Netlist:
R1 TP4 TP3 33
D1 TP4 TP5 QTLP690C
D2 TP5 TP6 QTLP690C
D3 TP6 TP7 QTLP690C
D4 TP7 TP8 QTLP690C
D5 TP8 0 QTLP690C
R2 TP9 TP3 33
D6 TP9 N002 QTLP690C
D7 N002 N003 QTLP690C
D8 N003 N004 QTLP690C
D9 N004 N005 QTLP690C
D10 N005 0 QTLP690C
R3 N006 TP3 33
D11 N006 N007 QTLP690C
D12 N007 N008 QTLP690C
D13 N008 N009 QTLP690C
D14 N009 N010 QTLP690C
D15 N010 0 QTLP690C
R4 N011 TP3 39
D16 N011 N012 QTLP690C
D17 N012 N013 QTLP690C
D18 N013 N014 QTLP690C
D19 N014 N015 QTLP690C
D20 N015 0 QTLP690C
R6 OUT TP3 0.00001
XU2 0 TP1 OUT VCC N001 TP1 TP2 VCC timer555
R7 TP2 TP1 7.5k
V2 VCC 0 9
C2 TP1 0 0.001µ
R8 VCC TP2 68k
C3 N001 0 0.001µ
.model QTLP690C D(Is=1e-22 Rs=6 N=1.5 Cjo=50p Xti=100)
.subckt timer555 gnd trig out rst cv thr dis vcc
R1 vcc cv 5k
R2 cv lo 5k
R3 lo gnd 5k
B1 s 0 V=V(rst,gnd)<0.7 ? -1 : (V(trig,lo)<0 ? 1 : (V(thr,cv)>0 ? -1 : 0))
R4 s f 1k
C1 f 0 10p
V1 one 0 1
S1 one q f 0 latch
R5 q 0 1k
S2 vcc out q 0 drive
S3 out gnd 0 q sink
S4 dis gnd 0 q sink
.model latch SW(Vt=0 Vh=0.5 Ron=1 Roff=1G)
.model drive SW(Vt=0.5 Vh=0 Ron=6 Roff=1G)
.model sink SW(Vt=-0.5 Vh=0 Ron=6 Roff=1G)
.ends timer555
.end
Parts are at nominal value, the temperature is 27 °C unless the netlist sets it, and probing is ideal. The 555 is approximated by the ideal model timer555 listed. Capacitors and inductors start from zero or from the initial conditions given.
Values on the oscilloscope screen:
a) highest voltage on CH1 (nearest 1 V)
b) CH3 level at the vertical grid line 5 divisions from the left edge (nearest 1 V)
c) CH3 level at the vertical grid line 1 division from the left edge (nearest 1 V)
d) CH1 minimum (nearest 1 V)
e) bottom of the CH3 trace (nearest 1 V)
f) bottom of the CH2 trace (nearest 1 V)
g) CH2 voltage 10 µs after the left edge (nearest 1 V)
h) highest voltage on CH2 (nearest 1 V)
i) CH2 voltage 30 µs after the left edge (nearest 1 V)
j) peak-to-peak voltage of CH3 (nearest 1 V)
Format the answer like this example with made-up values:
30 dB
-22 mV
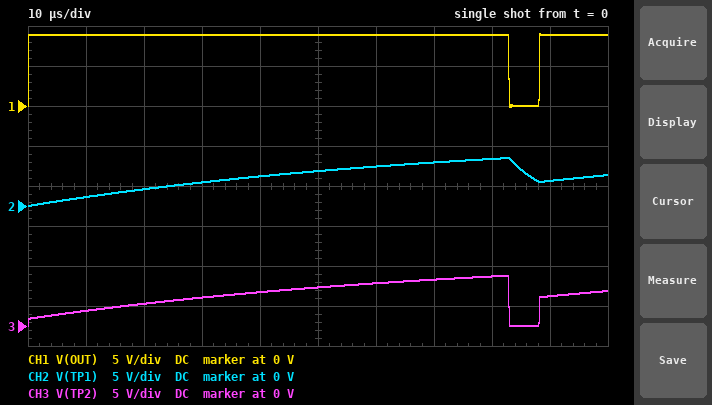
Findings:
9 V
5 V
2 V
0 V
0 V
0 V
1 V
6 V
3 V
6 V
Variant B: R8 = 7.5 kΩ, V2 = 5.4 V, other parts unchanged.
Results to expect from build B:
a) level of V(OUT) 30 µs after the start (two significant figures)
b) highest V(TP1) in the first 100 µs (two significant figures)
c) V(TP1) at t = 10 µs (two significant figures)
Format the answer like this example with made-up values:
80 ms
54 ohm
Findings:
5.4 V
3.6 V
2.6 V
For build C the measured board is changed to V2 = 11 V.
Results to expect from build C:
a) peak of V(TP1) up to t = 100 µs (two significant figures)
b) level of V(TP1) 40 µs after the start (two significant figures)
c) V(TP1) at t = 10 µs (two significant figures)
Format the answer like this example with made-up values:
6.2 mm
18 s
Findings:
7.3 V
4.5 V
1.4 V
